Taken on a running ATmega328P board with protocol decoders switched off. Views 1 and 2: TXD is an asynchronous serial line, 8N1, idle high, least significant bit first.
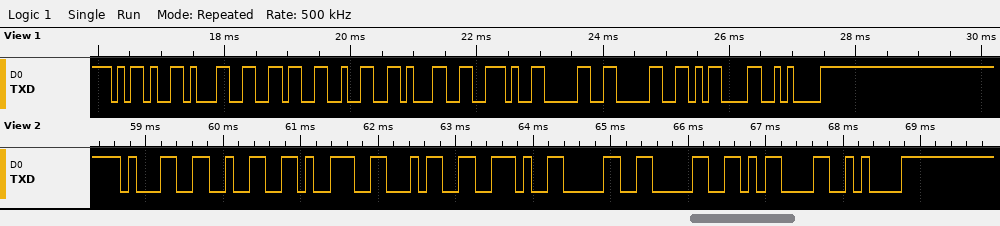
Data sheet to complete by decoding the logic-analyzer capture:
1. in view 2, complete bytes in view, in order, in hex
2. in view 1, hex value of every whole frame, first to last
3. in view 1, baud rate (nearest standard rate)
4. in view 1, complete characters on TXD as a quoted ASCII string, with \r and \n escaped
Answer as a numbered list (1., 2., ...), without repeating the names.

1. 31 32 39 34 2E 30 30 0D 0A
2. 0x2D 0x31 0x36 0x32 0x31 0x2E 0x30 0x30 0x0D 0x0A
3. 9600 baud
4. "-1621.00\r\n"
